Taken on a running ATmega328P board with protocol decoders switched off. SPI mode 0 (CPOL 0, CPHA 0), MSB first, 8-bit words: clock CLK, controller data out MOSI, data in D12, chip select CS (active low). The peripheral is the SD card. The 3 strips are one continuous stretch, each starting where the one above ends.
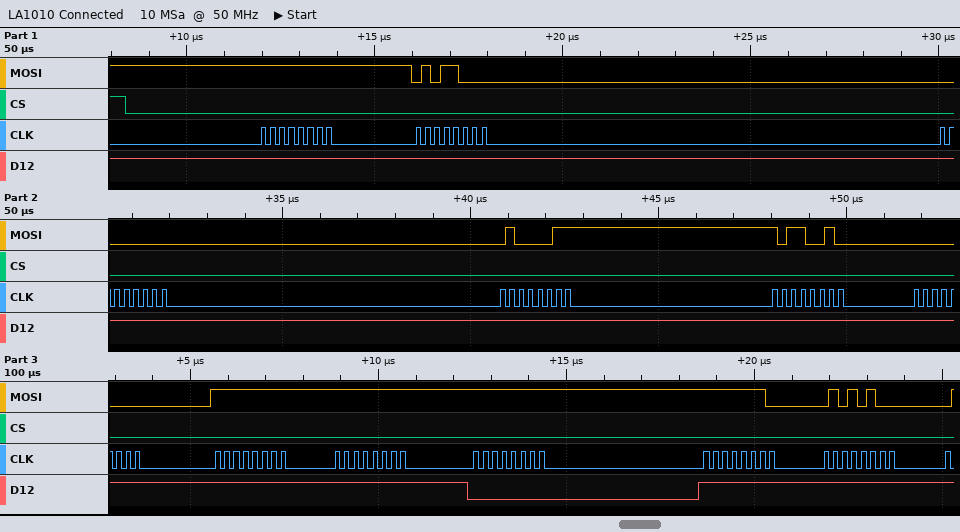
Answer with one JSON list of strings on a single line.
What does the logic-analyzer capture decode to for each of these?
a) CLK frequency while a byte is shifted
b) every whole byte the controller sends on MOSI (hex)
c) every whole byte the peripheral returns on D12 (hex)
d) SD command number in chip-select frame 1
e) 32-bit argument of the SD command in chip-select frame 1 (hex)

["4 MHz", "0xFF 0x58 0x00 0x43 0xB2 0x00 0xFF 0xFF 0xFF 0xFE 0x54", "0xFF 0xFF 0xFF 0xFF 0xFF 0xFF 0xFF 0xFF 0x00 0xFF 0xFF", "CMD24", "0x0043B200"]
